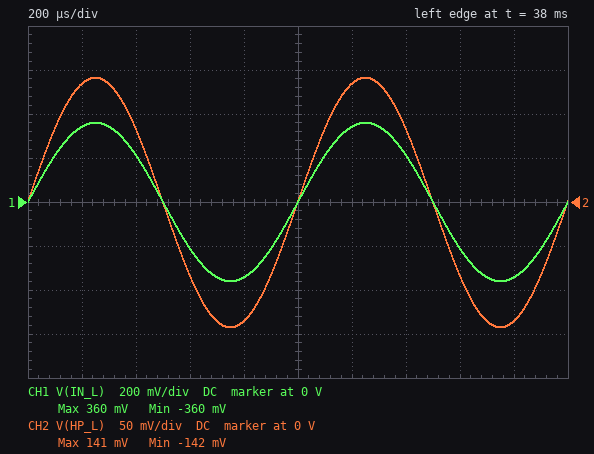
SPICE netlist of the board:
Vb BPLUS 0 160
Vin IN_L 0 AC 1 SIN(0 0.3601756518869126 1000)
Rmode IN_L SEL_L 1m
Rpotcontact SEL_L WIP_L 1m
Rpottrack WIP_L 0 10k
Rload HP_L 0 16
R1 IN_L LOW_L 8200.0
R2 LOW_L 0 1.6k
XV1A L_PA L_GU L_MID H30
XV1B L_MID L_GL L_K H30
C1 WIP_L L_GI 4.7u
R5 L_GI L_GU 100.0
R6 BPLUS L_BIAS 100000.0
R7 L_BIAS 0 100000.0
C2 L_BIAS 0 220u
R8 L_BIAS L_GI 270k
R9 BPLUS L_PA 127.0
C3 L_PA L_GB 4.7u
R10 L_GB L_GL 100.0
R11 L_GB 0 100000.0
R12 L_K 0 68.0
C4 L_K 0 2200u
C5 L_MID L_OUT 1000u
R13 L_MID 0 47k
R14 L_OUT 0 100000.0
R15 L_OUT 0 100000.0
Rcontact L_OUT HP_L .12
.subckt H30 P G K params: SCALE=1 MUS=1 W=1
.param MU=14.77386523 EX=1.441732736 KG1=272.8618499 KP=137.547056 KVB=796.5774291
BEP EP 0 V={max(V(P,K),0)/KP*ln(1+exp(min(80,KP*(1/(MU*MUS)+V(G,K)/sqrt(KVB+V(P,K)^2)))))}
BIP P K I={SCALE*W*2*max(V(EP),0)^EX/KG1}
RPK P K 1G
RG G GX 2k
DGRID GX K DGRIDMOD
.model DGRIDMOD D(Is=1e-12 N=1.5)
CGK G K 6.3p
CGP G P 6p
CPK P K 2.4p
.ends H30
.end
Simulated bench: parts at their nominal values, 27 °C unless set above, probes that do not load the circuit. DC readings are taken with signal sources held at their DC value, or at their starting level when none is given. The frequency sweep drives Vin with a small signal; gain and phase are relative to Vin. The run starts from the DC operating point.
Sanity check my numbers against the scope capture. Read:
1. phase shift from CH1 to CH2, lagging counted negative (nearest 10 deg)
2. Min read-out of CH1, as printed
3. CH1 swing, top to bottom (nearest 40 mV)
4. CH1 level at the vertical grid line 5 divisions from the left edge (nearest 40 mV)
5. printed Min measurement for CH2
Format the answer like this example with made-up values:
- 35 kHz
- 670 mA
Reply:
- 0 deg
- -360 mV
- 720 mV
- 0 V
- -142 mV
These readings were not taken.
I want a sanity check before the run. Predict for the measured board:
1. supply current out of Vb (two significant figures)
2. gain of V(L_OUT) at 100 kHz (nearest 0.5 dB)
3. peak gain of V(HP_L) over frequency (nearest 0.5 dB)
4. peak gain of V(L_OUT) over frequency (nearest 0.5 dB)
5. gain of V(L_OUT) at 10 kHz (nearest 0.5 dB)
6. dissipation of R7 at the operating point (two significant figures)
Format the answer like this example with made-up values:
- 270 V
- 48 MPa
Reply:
- 39 mA
- -8.0 dB
- -8.0 dB
- -8.0 dB
- -8.0 dB
- 64 mW
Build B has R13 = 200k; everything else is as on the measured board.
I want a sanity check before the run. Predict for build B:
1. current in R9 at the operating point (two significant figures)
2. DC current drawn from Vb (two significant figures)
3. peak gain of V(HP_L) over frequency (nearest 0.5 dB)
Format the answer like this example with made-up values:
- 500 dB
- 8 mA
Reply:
- 37 mA
- 38 mA
- -8.0 dB
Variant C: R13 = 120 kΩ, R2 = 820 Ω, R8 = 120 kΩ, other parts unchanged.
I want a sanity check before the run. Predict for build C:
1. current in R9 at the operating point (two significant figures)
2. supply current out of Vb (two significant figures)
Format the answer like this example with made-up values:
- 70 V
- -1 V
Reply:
- 37 mA
- 38 mA
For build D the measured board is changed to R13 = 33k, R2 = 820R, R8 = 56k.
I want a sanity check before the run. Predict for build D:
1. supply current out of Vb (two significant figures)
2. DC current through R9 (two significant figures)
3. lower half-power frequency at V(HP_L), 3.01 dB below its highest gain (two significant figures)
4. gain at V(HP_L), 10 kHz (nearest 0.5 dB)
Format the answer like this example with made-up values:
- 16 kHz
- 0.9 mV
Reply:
- 40 mA
- 39 mA
- 5.1 Hz
- -8.0 dB
